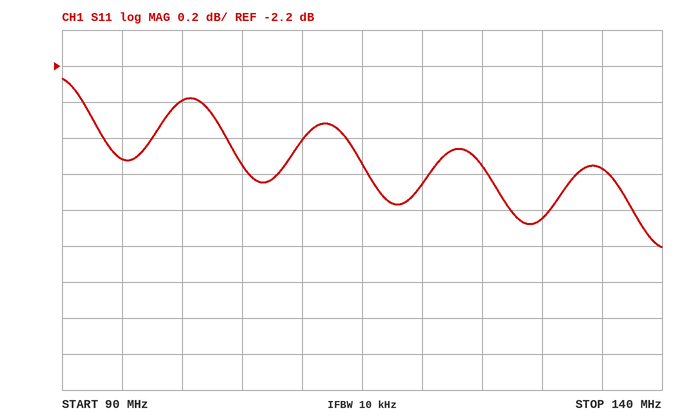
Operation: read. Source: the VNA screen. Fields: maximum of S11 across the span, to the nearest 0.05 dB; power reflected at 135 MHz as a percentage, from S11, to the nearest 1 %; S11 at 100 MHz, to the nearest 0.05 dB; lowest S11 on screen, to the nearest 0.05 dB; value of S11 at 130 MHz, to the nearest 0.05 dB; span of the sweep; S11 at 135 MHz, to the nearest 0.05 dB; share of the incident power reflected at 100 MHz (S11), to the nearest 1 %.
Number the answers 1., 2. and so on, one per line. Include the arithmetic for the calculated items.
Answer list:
1. -2.25 dB
2. 10^(-2.75/10) ≈ 53 %
3. -2.40 dB
4. -3.20 dB
5. -3.05 dB
6. 50 MHz
7. -2.75 dB
8. 10^(-2.4/10) ≈ 58 %
